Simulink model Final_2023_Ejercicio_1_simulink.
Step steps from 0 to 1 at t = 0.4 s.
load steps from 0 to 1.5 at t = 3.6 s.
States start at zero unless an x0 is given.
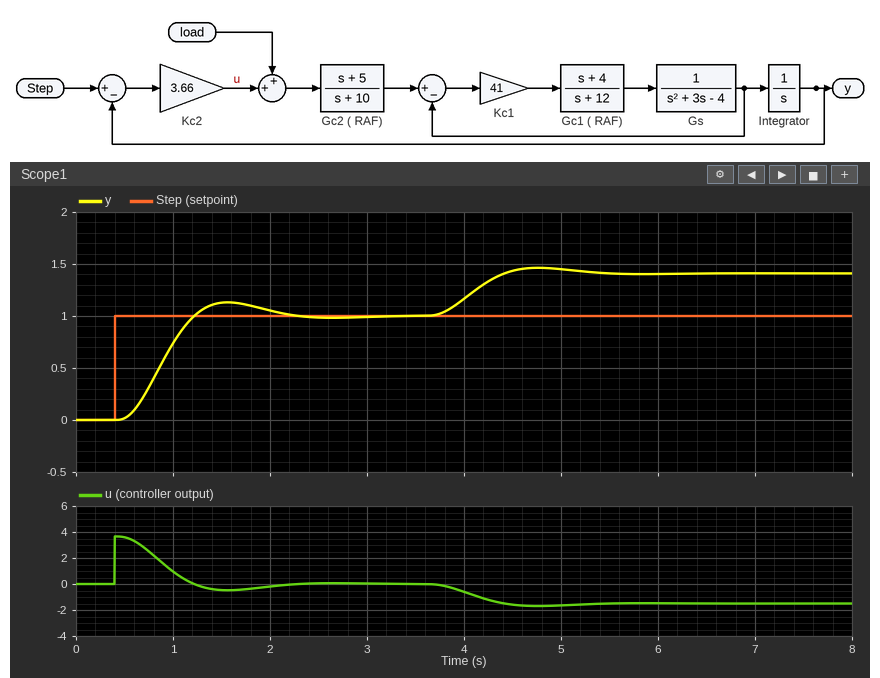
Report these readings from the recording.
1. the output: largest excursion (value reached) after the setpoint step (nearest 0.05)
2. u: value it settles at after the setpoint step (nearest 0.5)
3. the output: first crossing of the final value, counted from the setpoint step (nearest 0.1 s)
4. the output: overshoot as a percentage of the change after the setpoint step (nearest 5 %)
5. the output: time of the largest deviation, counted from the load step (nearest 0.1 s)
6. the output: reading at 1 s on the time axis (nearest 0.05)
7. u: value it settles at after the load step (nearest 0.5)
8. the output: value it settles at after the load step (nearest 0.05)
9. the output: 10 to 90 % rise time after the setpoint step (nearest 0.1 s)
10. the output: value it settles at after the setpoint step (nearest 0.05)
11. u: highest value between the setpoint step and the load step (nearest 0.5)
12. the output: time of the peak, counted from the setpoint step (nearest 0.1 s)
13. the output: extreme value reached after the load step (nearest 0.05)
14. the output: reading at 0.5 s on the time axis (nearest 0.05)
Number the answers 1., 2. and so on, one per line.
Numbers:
1. 1.15
2. 0.0
3. 0.8 s
4. 15 %
5. 1.2 s
6. 0.75
7. -1.5
8. 1.40
9. 0.5 s
10. 1.00
11. 3.5
12. 1.2 s
13. 1.45
14. 0.00
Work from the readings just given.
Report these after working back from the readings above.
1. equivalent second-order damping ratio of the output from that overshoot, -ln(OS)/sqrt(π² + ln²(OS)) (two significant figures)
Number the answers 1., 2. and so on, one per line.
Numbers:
1. 0.52
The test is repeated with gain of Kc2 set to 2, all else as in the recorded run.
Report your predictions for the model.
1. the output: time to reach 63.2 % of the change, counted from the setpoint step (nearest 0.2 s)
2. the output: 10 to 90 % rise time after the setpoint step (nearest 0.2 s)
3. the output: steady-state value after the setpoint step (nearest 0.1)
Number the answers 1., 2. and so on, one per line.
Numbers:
1. 0.8 s
2. 1.0 s
3. 1.0
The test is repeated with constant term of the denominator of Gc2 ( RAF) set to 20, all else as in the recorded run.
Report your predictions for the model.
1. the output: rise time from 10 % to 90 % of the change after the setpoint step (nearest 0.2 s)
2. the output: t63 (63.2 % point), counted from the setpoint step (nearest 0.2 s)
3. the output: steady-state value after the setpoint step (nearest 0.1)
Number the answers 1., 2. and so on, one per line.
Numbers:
1. 1.2 s
2. 0.8 s
3. 1.0
